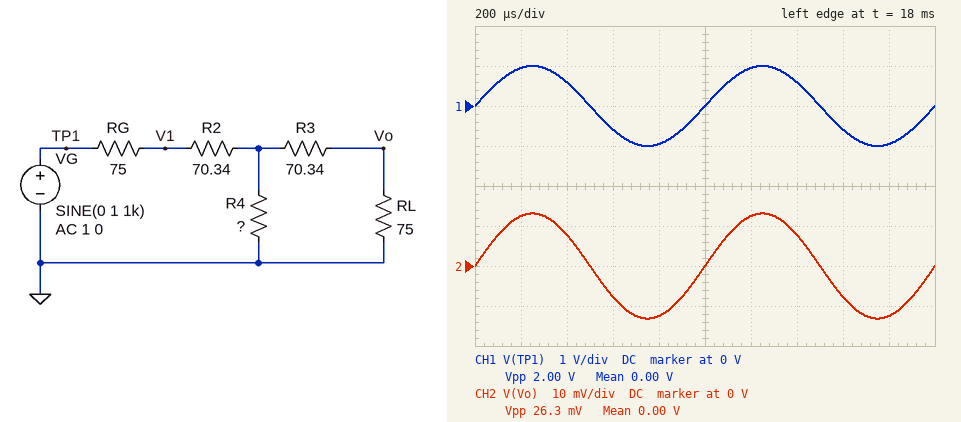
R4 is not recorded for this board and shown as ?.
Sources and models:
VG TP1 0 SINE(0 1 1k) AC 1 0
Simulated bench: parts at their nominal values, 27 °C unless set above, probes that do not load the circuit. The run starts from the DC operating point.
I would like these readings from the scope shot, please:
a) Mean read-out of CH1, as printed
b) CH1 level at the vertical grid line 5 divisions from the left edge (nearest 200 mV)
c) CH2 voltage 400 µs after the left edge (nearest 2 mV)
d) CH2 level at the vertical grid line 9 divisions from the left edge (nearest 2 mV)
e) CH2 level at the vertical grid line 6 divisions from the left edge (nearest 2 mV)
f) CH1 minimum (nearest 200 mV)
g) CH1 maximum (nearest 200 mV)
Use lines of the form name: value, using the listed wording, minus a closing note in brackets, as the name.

Mean read-out of CH1, as printed: 0.00 V
CH1 level at the vertical grid line 5 divisions from the left edge: 0 V
CH2 voltage 400 µs after the left edge: 8 mV
CH2 level at the vertical grid line 9 divisions from the left edge: -12 mV
CH2 level at the vertical grid line 6 divisions from the left edge: 12 mV
CH1 minimum: -1.0 V
CH1 maximum: 1.0 V
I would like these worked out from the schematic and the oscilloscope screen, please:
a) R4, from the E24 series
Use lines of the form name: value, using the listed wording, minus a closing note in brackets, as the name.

R4, from the E24 series: 3.9 Ω
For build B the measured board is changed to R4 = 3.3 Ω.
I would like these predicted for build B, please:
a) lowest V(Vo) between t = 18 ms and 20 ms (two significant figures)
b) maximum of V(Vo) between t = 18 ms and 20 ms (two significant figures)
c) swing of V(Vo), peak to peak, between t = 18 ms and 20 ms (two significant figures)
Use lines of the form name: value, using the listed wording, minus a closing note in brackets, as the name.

lowest V(Vo) between t = 18 ms and 20 ms: -11 mV
maximum of V(Vo) between t = 18 ms and 20 ms: 11 mV
swing of V(Vo), peak to peak, between t = 18 ms and 20 ms: 22 mV
